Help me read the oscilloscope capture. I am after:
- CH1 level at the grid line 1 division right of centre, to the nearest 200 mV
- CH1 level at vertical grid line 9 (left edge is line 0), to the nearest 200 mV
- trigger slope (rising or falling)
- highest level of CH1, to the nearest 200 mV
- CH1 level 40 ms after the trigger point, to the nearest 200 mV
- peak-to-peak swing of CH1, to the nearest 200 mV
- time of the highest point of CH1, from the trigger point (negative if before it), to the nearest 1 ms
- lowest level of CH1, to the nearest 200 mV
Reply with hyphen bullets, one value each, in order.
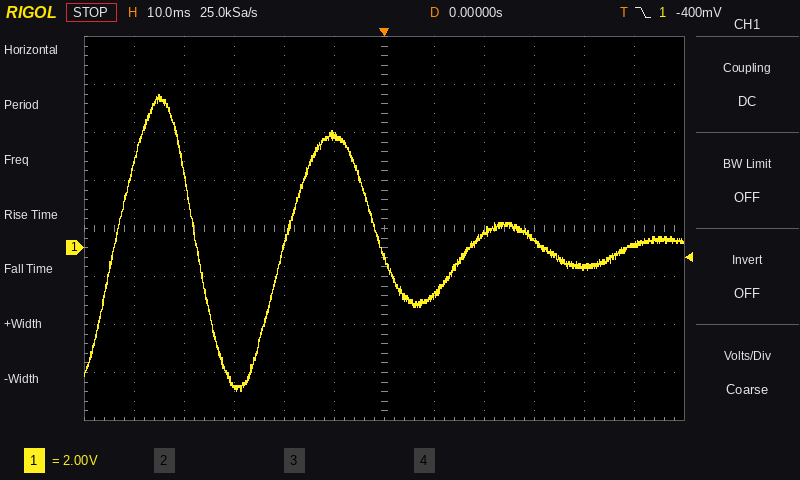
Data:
- -2.0 V
- 400 mV
- falling
- 6.4 V
- -800 mV
- 12.4 V
- -45 ms
- -6.0 V
